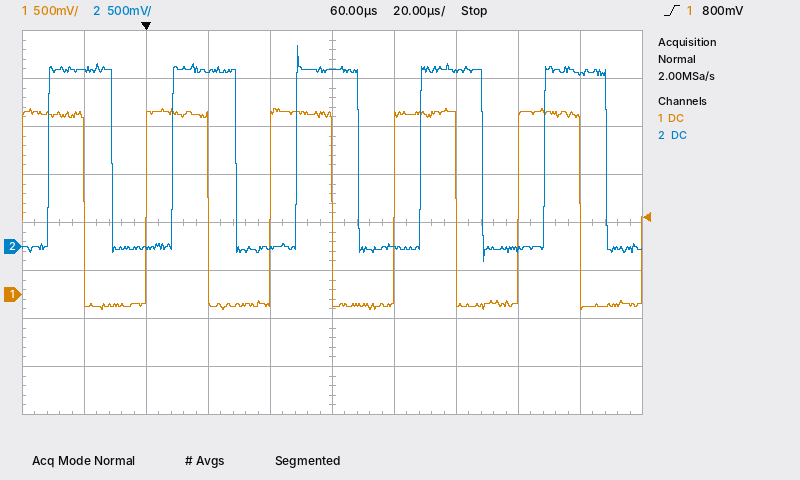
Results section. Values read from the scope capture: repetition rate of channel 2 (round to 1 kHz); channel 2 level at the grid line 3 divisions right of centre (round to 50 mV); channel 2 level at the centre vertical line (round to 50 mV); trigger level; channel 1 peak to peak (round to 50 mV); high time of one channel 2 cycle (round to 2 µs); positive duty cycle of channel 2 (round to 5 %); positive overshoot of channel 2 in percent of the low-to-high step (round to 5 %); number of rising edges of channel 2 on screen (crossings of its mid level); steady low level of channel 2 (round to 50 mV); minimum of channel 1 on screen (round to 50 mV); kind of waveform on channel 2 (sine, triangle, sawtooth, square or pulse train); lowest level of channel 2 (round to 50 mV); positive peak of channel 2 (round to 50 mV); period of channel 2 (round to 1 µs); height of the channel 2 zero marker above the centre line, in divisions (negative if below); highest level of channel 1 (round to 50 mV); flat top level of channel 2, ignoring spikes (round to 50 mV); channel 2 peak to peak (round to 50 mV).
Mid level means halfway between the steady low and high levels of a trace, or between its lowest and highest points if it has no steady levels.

25 kHz
-50 mV
1.85 V
800 mV
2.10 V
20 µs
50 %
15 %
5
0 mV
-150 mV
square
-150 mV
2.10 V
40 µs
-0.5 div
1.95 V
1.85 V
2.25 V
